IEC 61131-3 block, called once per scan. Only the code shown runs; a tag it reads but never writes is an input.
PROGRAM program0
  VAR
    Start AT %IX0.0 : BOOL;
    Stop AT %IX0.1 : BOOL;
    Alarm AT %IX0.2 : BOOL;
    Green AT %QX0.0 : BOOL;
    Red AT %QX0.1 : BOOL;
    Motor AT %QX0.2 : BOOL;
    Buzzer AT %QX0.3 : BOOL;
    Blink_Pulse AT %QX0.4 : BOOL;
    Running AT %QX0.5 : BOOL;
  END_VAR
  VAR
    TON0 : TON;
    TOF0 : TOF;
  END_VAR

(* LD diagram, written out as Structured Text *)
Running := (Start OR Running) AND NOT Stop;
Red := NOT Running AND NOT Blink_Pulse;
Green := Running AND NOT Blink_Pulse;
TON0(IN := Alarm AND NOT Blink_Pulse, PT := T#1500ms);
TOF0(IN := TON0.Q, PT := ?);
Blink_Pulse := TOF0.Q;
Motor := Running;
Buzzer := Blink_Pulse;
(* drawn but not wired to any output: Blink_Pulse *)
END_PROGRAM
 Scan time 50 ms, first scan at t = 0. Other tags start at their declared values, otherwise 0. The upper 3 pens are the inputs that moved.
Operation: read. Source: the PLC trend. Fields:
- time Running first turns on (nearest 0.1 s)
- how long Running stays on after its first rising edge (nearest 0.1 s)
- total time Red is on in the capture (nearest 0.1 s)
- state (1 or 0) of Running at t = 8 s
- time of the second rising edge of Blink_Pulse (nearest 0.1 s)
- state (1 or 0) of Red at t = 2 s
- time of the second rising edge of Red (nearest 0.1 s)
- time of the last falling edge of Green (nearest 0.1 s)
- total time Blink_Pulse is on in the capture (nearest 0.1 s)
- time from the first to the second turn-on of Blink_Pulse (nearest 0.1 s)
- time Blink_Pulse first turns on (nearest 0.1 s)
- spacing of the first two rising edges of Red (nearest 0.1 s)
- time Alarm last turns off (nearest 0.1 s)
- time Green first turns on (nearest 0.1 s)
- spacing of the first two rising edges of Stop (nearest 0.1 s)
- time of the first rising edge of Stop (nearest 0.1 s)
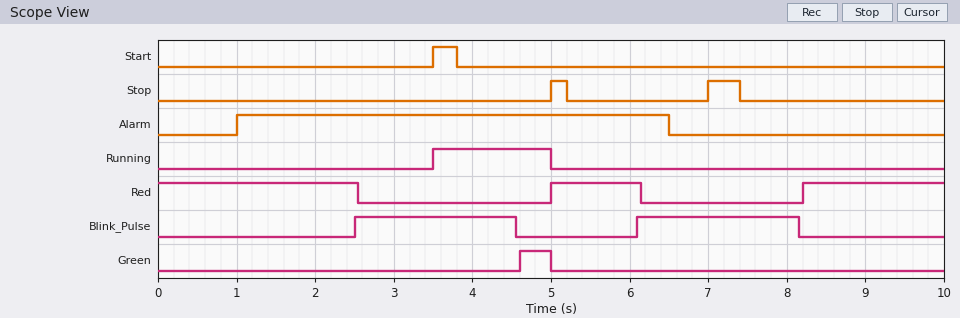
3.5 s
1.5 s
5.5 s
0
6.1 s
1
8.2 s
5.0 s
4.1 s
3.6 s
2.5 s
3.2 s
6.5 s
4.6 s
2.0 s
5.0 s
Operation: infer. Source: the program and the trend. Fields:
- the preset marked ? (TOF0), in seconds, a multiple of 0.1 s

2.0 s
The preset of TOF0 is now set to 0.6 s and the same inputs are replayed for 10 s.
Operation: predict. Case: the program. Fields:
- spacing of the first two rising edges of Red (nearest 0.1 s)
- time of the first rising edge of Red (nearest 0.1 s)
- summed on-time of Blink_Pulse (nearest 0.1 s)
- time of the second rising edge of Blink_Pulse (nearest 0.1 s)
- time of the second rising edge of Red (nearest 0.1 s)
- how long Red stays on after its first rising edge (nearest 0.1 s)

2.2 s
3.2 s
1.3 s
4.7 s
5.4 s
0.3 s
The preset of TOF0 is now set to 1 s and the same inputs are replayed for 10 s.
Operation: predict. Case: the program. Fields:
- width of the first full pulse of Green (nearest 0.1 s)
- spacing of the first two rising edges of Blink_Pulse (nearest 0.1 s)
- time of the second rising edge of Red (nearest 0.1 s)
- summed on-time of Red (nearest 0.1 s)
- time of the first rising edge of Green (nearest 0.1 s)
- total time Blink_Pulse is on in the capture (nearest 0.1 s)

1.4 s
2.6 s
6.2 s
6.5 s
3.6 s
2.1 s
